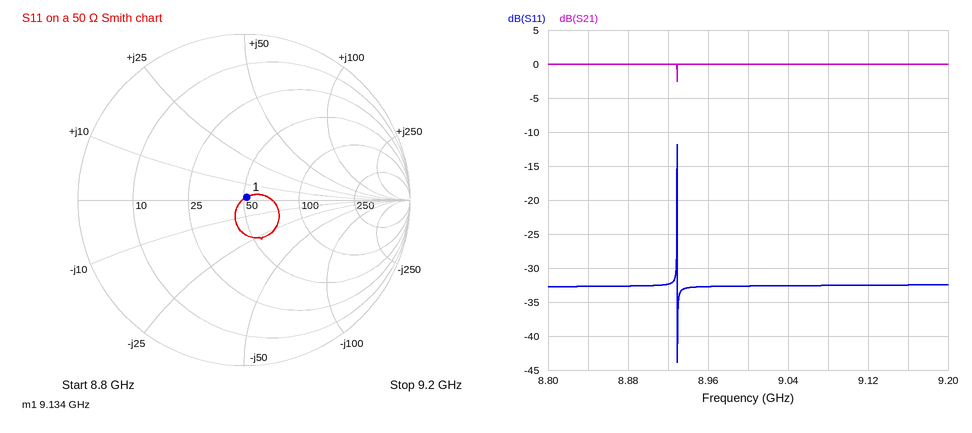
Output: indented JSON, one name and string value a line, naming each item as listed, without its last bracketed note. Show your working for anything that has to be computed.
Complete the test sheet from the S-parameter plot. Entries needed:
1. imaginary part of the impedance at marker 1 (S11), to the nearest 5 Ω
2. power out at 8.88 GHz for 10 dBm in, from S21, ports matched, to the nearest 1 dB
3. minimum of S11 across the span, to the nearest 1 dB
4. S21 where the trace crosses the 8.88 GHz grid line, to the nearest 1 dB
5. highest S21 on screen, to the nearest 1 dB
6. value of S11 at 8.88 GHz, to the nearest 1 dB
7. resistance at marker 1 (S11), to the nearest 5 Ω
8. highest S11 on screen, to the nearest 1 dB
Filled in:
{
  "imaginary part of the impedance at marker 1 (S11), to the nearest 5 Ω": "0 Ω",
  "power out at 8.88 GHz for 10 dBm in, from S21, ports matched, to the nearest 1 dB": "10 dBm + (0 dB) = 10 dBm",
  "minimum of S11 across the span, to the nearest 1 dB": "-44 dB",
  "S21 where the trace crosses the 8.88 GHz grid line, to the nearest 1 dB": "0 dB",
  "highest S21 on screen, to the nearest 1 dB": "0 dB",
  "value of S11 at 8.88 GHz, to the nearest 1 dB": "-33 dB",
  "resistance at marker 1 (S11), to the nearest 5 Ω": "50 Ω",
  "highest S11 on screen, to the nearest 1 dB": "-12 dB"
}
